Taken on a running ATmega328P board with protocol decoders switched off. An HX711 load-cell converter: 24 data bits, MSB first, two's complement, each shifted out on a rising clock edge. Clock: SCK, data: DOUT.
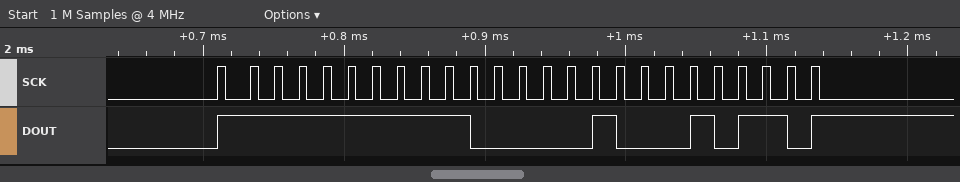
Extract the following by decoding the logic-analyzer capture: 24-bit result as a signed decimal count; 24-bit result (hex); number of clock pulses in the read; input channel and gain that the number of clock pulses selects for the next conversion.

-16106
0xFFC116
25
channel A, gain 128
